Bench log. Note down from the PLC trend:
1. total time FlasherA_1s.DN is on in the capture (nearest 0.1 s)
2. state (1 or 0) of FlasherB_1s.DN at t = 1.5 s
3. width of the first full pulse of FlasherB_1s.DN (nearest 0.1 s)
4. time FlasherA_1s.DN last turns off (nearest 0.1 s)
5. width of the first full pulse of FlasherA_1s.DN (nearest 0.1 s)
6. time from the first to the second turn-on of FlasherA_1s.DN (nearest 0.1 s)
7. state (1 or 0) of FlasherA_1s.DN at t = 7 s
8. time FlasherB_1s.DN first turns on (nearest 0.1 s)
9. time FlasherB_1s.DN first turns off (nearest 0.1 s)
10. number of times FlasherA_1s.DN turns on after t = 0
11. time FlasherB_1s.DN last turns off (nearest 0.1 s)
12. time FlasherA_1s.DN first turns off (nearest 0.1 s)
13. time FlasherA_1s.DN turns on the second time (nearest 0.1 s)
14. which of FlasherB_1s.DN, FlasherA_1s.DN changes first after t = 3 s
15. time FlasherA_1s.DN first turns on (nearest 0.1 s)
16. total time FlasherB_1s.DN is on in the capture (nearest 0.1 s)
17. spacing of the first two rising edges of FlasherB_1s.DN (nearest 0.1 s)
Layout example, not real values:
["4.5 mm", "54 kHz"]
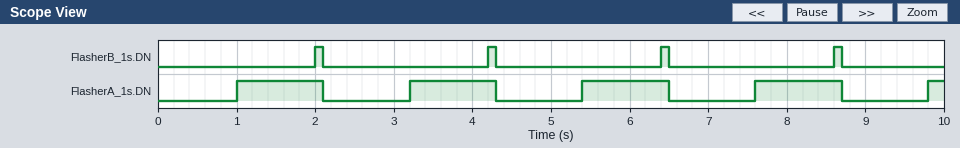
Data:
["4.6 s", "0", "0.1 s", "8.7 s", "1.1 s", "2.2 s", "0", "2.0 s", "2.1 s", "5", "8.7 s", "2.1 s", "3.2 s", "FlasherA_1s.DN", "1.0 s", "0.4 s", "2.2 s"]
